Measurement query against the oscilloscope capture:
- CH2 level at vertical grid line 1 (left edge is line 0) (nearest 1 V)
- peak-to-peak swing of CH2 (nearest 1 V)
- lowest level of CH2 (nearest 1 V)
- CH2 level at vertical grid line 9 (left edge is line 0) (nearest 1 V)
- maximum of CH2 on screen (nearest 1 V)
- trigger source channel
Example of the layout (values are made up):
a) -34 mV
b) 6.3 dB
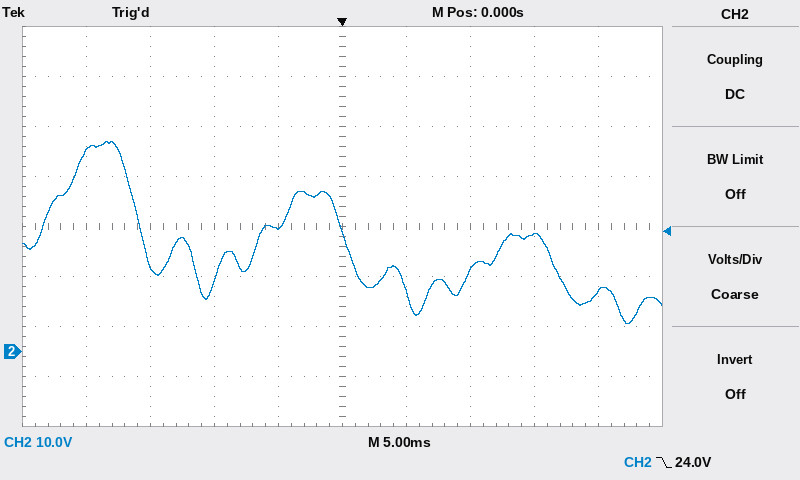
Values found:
a) 40 V
b) 36 V
c) 6 V
d) 12 V
e) 42 V
f) CH2
